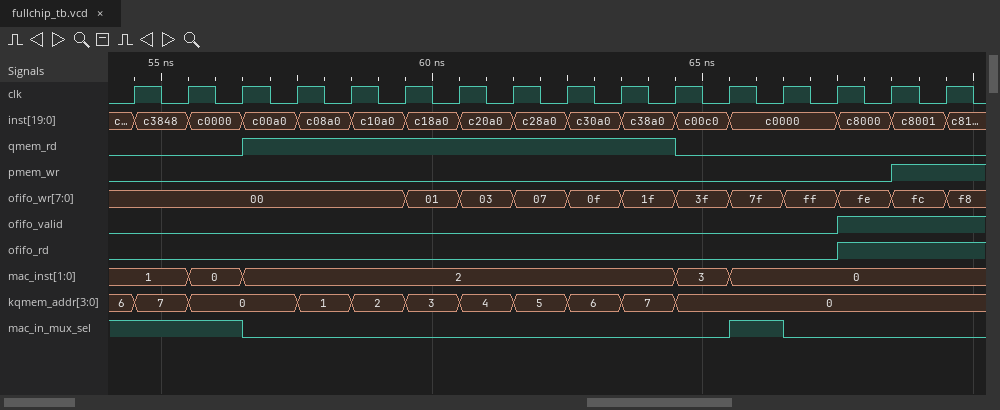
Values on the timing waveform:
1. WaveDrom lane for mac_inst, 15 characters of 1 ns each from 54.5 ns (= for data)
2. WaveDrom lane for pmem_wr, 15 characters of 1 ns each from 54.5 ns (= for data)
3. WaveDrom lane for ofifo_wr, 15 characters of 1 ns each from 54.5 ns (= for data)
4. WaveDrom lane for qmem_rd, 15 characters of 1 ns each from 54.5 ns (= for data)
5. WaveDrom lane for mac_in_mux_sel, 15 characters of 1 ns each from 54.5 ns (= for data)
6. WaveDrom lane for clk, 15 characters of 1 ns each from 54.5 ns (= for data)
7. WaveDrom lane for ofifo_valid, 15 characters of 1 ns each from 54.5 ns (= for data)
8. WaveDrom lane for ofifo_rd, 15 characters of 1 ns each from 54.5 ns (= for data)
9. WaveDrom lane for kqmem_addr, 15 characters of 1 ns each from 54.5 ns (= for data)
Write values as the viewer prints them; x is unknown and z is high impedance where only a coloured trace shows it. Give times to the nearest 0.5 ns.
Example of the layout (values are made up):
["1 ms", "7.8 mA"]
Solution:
["{name: 'mac_inst', wave: '===.......==...', data: '1 0 2 3 0'}", "{name: 'pmem_wr', wave: '0.............1'}", "{name: 'ofifo_wr', wave: '=....==========', data: '00 01 03 07 0f 1f 3f 7f ff fe fc'}", "{name: 'qmem_rd', wave: '0.1.......0....'}", "{name: 'mac_in_mux_sel', wave: '1.0........10..'}", "{name: 'clk', wave: 'p..............'}", "{name: 'ofifo_valid', wave: '0............1.'}", "{name: 'ofifo_rd', wave: '0............1.'}", "{name: 'kqmem_addr', wave: '==.========....', data: '7 0 1 2 3 4 5 6 7 0'}"]
